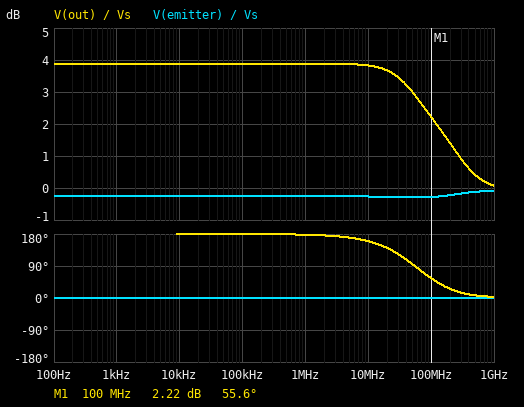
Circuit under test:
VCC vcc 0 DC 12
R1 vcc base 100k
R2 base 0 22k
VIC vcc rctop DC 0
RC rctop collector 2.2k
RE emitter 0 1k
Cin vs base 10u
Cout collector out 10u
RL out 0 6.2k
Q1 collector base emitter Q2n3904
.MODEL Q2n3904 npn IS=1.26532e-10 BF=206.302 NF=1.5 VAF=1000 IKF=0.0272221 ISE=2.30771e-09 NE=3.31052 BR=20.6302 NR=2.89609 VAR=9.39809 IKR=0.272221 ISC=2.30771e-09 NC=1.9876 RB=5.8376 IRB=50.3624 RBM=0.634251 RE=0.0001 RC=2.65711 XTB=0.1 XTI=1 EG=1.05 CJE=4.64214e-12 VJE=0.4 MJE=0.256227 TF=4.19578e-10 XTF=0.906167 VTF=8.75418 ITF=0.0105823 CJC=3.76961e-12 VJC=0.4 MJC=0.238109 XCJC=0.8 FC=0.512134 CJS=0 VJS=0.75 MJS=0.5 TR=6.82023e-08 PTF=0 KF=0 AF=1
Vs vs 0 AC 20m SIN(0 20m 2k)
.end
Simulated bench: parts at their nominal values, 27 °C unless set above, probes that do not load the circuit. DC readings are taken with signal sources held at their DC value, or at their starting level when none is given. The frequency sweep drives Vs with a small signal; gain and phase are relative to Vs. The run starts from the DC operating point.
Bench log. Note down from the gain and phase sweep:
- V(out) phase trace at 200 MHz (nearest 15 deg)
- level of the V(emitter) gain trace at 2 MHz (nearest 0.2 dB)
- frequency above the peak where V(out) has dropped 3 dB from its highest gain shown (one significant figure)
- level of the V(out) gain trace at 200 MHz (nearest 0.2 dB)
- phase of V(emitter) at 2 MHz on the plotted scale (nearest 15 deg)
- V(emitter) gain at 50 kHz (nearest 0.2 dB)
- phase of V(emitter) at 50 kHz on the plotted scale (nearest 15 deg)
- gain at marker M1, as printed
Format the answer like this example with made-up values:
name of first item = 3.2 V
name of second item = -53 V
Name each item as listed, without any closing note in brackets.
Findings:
V(out) phase trace at 200 MHz = 30 deg
level of the V(emitter) gain trace at 2 MHz = -0.2 dB
frequency above the peak where V(out) has dropped 3 dB from its highest gain shown = 300 MHz
level of the V(out) gain trace at 200 MHz = 1.4 dB
phase of V(emitter) at 2 MHz on the plotted scale = 0 deg
V(emitter) gain at 50 kHz = -0.2 dB
phase of V(emitter) at 50 kHz on the plotted scale = 0 deg
gain at marker M1, as printed = 2.22 dB
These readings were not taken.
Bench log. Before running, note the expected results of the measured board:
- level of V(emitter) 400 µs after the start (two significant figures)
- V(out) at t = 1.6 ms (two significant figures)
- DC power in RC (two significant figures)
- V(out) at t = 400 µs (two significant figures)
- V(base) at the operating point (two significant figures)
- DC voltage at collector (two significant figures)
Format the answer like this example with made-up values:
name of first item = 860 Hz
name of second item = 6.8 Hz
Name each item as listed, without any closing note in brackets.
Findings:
level of V(emitter) 400 µs after the start = 1.3 V
V(out) at t = 1.6 ms = -30 mV
DC power in RC = 3.9 mW
V(out) at t = 400 µs = 30 mV
V(base) at the operating point = 2.0 V
DC voltage at collector = 9.1 V
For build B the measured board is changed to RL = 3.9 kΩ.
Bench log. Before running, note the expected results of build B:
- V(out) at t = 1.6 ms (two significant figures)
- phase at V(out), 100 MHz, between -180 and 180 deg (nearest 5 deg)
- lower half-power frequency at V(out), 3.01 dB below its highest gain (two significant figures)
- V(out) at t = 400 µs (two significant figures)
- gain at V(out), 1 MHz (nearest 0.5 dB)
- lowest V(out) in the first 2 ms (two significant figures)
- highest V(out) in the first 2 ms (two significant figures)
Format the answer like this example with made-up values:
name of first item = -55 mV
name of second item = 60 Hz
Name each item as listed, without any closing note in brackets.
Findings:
V(out) at t = 1.6 ms = -26 mV
phase at V(out), 100 MHz, between -180 and 180 deg = 60 deg
lower half-power frequency at V(out), 3.01 dB below its highest gain = 2.9 Hz
V(out) at t = 400 µs = 26 mV
gain at V(out), 1 MHz = 2.5 dB
lowest V(out) in the first 2 ms = -27 mV
highest V(out) in the first 2 ms = 27 mV
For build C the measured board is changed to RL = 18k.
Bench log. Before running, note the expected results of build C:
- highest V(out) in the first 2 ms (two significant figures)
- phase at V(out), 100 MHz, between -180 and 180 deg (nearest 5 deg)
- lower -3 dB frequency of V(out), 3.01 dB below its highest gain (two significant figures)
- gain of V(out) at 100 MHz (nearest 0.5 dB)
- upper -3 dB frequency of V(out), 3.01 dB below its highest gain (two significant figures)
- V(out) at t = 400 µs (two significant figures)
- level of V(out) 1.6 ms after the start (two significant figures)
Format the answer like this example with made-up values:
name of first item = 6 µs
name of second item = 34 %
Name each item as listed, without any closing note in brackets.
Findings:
highest V(out) in the first 2 ms = 38 mV
phase at V(out), 100 MHz, between -180 and 180 deg = 50 deg
lower -3 dB frequency of V(out), 3.01 dB below its highest gain = 1.4 Hz
gain of V(out) at 100 MHz = 2.5 dB
upper -3 dB frequency of V(out), 3.01 dB below its highest gain = 100 MHz
V(out) at t = 400 µs = 36 mV
level of V(out) 1.6 ms after the start = -36 mV
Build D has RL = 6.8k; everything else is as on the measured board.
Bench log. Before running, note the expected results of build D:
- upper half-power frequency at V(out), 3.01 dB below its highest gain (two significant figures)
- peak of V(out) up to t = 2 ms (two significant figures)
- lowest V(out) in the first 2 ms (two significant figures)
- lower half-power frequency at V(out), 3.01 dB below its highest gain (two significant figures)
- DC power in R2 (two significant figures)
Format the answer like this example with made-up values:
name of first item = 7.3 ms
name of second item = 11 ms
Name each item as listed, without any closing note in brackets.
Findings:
upper half-power frequency at V(out), 3.01 dB below its highest gain = 260 MHz
peak of V(out) up to t = 2 ms = 32 mV
lowest V(out) in the first 2 ms = -32 mV
lower half-power frequency at V(out), 3.01 dB below its highest gain = 2.2 Hz
DC power in R2 = 180 µW
